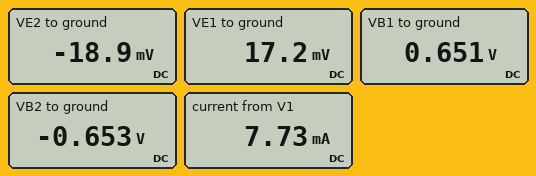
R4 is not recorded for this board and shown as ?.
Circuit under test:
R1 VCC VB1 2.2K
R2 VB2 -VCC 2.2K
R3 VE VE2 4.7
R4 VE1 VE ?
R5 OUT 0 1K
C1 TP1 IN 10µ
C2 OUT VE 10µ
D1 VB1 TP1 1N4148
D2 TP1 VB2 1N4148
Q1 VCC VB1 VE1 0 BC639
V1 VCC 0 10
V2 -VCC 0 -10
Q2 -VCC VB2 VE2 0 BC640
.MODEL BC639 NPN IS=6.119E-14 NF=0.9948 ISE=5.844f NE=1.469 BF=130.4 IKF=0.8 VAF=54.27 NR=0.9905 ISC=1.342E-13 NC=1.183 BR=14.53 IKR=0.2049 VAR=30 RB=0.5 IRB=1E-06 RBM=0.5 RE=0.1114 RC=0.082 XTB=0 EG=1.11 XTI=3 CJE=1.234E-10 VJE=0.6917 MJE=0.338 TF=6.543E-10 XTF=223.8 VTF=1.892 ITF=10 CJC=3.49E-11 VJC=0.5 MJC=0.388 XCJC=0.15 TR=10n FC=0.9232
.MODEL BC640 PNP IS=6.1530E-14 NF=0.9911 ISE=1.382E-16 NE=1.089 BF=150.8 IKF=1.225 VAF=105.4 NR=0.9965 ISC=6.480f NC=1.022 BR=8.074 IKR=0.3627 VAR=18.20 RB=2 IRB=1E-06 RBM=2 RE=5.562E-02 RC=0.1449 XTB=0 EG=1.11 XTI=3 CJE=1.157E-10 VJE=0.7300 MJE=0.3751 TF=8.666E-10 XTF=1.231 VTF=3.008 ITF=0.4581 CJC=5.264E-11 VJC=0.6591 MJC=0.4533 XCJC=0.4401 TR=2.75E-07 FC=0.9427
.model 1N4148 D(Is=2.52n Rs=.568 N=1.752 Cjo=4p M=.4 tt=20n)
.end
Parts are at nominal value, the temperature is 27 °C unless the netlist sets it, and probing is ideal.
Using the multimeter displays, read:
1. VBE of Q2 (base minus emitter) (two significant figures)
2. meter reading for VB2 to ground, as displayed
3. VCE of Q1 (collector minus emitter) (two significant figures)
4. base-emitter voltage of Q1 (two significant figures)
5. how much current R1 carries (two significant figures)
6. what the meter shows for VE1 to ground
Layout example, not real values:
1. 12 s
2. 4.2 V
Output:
1. -630 mV
2. -0.653 V
3. 10 V
4. 630 mV
5. 4.2 mA
6. 17.2 mV
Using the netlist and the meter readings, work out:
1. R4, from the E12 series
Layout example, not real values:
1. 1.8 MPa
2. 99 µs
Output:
1. 5.6 Ω
